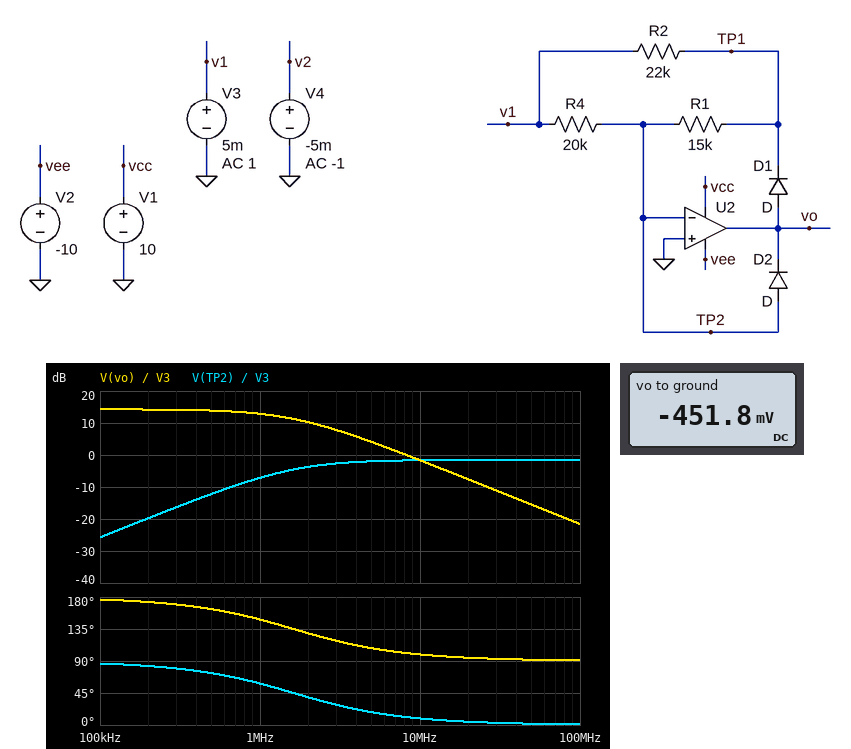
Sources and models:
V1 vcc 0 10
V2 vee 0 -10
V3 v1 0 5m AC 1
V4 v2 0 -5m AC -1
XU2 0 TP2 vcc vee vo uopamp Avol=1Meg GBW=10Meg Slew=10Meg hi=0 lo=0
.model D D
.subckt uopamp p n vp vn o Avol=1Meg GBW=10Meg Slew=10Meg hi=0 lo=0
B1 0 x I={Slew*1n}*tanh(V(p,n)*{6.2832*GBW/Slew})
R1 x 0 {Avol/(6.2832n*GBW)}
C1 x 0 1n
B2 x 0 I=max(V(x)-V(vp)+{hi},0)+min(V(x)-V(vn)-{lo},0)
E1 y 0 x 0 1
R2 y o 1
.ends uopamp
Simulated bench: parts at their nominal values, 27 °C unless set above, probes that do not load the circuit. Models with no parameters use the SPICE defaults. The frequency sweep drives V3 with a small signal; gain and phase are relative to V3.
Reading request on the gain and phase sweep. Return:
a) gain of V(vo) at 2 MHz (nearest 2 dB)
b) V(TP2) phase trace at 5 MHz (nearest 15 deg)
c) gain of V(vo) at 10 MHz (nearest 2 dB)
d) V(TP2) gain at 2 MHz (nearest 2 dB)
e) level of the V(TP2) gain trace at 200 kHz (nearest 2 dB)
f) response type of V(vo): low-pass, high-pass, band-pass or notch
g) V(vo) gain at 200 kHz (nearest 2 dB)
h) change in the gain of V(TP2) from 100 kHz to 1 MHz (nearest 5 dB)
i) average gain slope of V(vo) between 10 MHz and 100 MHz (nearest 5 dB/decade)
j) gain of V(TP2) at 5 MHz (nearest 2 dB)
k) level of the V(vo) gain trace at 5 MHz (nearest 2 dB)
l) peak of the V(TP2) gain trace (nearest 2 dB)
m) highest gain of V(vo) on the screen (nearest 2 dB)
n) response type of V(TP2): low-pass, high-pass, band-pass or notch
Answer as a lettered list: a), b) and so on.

a) 10 dB
b) 15 deg
c) -2 dB
d) -4 dB
e) -20 dB
f) low-pass
g) 14 dB
h) 20 dB
i) -20 dB/decade
j) -2 dB
k) 4 dB
l) -2 dB
m) 14 dB
n) high-pass
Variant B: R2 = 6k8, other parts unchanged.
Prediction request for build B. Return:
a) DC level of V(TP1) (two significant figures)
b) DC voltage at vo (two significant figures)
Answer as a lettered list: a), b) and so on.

a) 3.4 mV
b) -460 mV
